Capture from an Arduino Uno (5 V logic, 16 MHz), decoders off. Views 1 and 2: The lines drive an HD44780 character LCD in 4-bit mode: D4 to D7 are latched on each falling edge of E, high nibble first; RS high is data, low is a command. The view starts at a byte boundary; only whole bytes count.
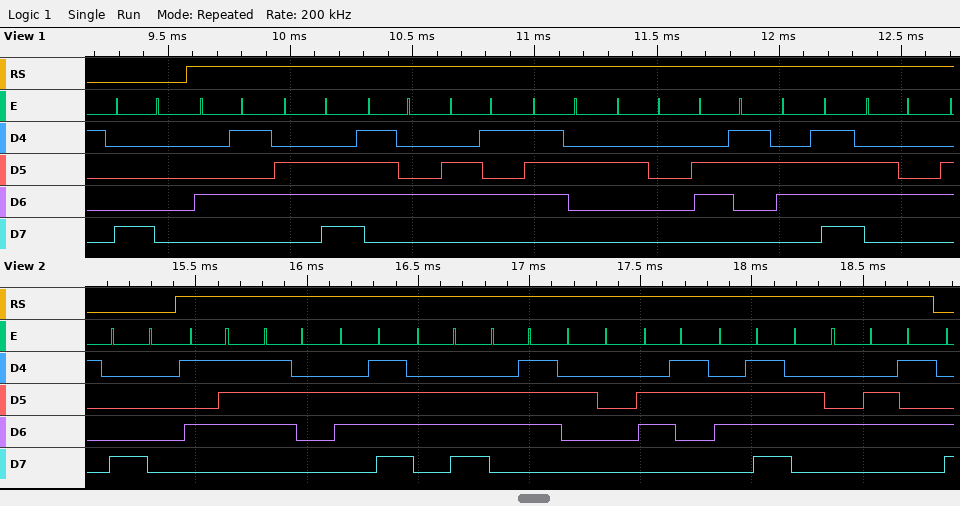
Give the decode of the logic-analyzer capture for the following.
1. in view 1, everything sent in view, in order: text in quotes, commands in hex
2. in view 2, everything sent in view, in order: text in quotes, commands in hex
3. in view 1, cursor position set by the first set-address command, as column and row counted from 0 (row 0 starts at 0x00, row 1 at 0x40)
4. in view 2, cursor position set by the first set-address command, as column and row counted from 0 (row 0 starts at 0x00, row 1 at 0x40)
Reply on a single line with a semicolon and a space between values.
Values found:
0x80 "Enter cod"; 0x80 "Wrong code"; column 0, row 0; column 0, row 0
